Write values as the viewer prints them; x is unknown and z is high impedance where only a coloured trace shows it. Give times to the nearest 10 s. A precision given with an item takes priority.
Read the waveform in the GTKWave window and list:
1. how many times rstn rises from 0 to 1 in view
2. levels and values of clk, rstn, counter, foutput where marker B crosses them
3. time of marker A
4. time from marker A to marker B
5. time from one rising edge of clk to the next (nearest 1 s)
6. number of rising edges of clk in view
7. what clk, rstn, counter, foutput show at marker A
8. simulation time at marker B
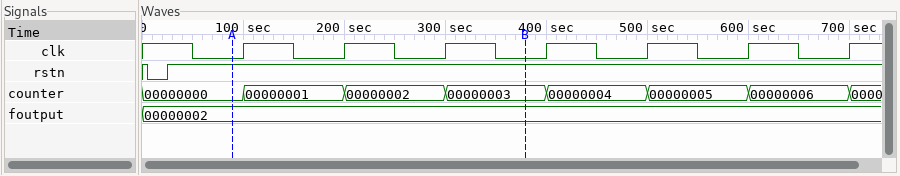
1
clk=0, rstn=1, counter=00000003, foutput=00000002
90 s
290 s
100 s
7
clk=0, rstn=1, counter=00000000, foutput=00000002
380 s
